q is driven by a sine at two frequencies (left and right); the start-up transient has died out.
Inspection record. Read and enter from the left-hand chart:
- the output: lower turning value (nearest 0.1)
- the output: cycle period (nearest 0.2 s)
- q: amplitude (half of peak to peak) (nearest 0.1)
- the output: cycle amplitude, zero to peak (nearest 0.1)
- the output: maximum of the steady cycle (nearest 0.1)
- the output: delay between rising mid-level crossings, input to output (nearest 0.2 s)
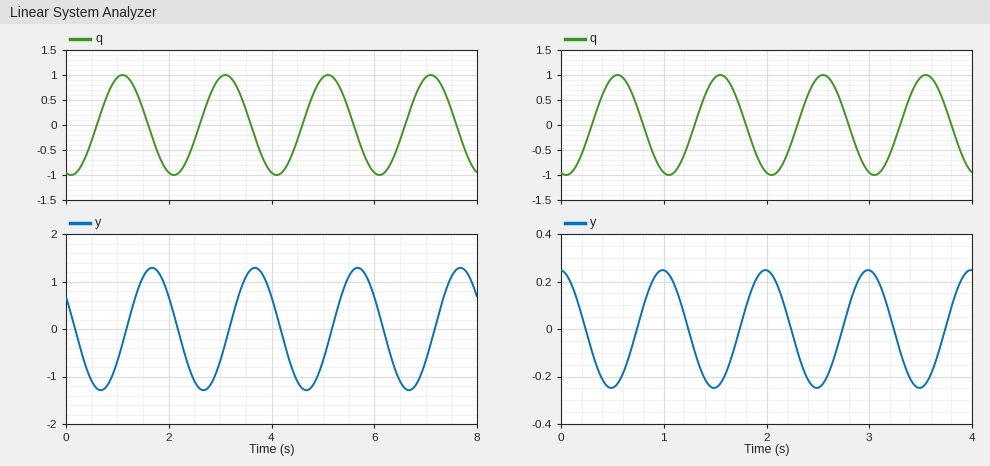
-1.3
2.0 s
1.0
1.3
1.3
0.6 s
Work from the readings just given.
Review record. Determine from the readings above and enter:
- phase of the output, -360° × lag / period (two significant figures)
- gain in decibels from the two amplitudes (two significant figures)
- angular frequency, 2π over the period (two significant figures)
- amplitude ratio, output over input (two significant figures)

-110°
2.3 dB
3.1 rad/s
1.3
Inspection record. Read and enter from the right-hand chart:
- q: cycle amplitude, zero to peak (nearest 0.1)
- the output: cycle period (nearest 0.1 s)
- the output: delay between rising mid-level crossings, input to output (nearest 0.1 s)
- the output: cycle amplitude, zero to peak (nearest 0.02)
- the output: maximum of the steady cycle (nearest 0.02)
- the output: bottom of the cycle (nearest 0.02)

1.0
1.0 s
0.4 s
0.24
0.24
-0.24
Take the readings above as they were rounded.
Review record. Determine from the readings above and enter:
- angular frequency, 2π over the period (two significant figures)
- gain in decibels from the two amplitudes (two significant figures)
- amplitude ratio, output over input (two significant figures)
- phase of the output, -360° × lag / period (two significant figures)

6.3 rad/s
-12 dB
0.24
-140°
